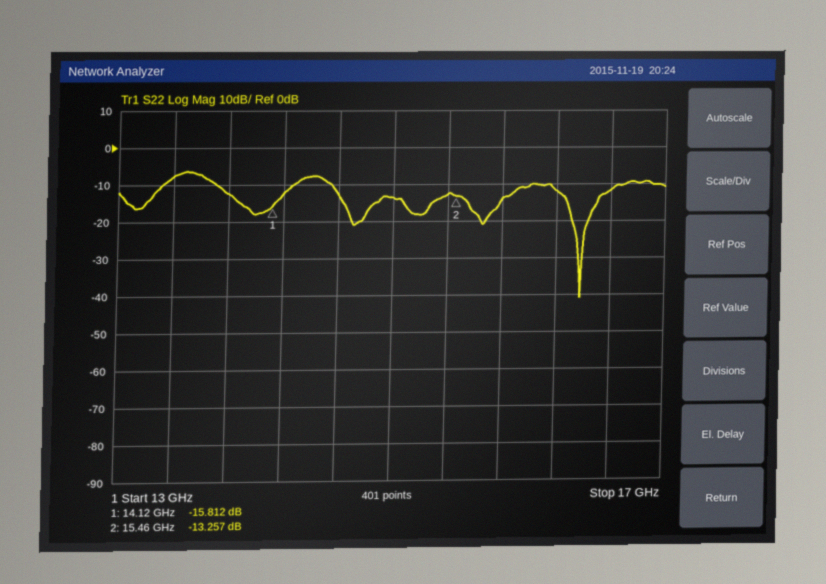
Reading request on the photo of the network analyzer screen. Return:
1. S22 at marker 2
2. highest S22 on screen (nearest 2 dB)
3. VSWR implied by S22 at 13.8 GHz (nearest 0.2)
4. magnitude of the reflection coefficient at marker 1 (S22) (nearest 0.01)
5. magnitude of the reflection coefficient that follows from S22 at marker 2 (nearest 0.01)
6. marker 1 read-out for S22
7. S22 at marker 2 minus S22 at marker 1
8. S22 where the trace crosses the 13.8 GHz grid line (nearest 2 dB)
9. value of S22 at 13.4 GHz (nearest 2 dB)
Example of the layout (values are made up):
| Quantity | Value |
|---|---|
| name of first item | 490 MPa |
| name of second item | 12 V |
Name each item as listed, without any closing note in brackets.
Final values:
| Quantity | Value |
|---|---|
| S22 at marker 2 | -13.257 dB |
| highest S22 on screen | -6 dB |
| VSWR implied by S22 at 13.8 GHz | 1.6 |
| magnitude of the reflection coefficient at marker 1 (S22) | 0.16 |
| magnitude of the reflection coefficient that follows from S22 at marker 2 | 0.22 |
| marker 1 read-out for S22 | -15.812 dB |
| S22 at marker 2 minus S22 at marker 1 | 2.555 dB |
| S22 where the trace crosses the 13.8 GHz grid line | -12 dB |
| value of S22 at 13.4 GHz | -8 dB |
